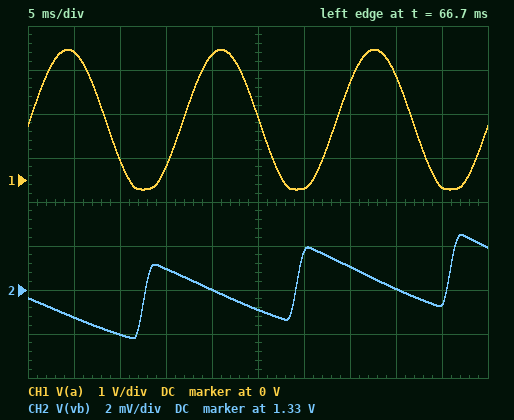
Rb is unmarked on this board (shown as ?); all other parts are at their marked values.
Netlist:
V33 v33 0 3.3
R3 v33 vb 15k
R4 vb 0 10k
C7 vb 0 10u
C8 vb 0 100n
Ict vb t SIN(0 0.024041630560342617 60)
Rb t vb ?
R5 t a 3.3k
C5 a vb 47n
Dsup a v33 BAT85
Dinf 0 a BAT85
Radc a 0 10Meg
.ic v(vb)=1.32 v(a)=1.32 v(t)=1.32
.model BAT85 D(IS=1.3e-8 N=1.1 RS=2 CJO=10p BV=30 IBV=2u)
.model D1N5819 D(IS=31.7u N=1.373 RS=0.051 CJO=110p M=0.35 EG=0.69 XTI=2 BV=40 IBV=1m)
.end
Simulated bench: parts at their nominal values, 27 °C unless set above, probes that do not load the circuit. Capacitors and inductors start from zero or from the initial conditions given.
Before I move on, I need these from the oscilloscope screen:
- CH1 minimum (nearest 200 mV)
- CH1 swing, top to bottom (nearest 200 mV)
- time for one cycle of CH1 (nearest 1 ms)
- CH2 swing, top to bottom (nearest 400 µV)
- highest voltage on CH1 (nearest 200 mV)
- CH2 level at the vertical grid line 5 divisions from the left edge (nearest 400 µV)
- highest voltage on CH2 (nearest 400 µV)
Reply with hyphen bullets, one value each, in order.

- -200 mV
- 3.2 V
- 17 ms
- 4.8 mV
- 3.0 V
- 1.3292 V
- 1.3324 V
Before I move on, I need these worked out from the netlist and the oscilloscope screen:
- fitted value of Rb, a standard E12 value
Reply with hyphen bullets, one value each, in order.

- 68 Ω
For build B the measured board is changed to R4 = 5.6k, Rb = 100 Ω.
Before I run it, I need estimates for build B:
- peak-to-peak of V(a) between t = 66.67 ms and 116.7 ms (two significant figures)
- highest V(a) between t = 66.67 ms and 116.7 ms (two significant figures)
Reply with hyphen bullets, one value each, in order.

- 3.8 V
- 3.5 V
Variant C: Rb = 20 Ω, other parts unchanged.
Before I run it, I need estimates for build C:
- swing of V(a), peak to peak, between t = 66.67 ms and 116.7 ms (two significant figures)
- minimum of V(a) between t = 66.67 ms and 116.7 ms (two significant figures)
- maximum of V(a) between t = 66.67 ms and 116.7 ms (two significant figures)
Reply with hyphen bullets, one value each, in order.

- 960 mV
- 840 mV
- 1.8 V
